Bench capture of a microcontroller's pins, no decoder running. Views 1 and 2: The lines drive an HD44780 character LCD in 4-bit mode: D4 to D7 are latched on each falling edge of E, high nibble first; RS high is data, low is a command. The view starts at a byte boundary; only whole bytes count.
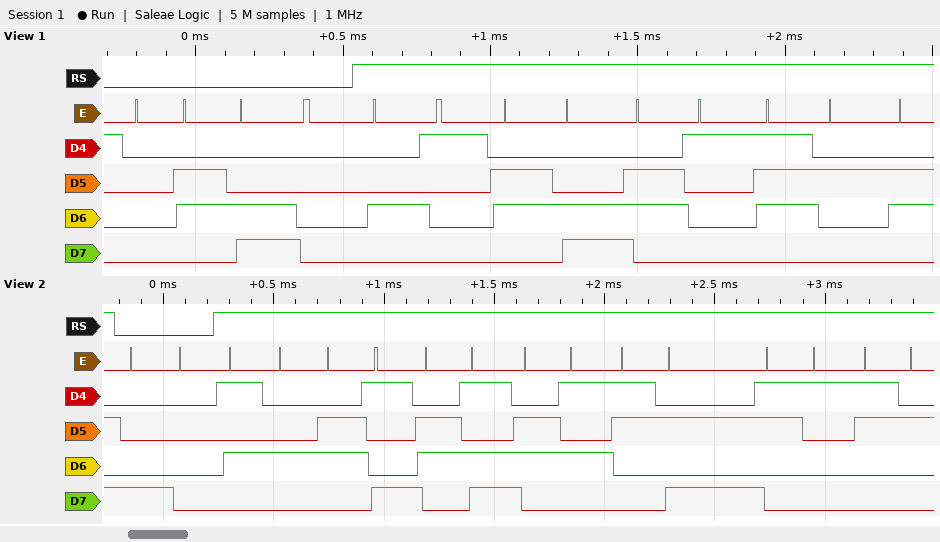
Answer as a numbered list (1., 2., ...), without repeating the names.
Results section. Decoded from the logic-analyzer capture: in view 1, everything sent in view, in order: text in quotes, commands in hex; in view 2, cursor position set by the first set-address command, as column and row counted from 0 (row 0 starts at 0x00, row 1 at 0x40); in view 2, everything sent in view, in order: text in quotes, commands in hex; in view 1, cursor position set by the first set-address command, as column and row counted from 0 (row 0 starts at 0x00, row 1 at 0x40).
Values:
1. 0x06 0xC0 "Alar"
2. column 0, row 0
3. 0x80 "Time:12"
4. column 0, row 1
